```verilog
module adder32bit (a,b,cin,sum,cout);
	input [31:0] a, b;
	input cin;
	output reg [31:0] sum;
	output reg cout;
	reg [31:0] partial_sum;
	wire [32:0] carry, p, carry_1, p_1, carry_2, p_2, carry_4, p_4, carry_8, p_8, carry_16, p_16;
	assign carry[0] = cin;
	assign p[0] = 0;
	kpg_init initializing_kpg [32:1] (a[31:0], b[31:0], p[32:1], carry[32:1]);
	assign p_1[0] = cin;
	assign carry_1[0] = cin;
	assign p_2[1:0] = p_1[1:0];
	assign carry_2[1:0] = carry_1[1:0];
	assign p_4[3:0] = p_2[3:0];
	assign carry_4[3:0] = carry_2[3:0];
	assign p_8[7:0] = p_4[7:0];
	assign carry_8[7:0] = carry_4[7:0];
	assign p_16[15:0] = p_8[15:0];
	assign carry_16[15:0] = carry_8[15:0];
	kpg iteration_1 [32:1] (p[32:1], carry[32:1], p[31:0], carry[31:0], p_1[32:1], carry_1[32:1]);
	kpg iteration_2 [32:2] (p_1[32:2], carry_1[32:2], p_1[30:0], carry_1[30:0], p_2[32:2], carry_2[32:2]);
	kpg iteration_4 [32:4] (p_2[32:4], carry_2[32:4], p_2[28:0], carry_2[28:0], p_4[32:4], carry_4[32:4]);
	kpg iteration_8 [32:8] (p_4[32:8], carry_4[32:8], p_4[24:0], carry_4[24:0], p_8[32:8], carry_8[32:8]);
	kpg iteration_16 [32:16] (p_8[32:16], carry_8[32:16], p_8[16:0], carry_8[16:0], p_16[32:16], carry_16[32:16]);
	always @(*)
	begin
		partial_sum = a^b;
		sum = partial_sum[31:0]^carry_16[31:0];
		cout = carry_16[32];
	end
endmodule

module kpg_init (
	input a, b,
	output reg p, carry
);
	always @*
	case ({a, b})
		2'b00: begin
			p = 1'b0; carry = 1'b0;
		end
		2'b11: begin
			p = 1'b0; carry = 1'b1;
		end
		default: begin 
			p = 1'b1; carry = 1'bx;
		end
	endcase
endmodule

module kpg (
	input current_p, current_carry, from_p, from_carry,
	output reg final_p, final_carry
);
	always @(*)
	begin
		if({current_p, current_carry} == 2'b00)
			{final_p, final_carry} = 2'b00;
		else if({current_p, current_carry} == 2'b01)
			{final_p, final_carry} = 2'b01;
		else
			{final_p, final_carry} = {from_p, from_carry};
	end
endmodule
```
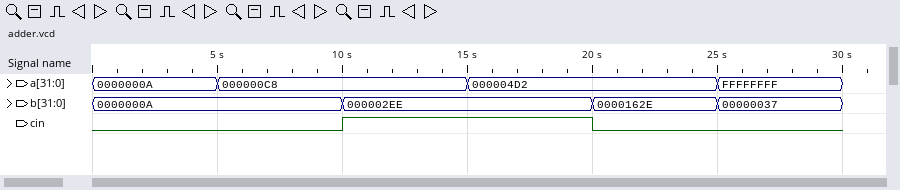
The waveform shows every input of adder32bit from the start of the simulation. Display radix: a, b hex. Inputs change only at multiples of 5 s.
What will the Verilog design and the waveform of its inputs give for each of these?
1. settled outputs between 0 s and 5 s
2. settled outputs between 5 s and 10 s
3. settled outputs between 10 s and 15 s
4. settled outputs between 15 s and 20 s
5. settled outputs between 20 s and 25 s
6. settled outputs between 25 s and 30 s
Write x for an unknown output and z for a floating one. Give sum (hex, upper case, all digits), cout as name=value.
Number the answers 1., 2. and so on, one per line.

1. sum=00000014, cout=0
2. sum=000000D2, cout=0
3. sum=000003B7, cout=0
4. sum=000007C1, cout=0
5. sum=00001B00, cout=0
6. sum=00000036, cout=1
